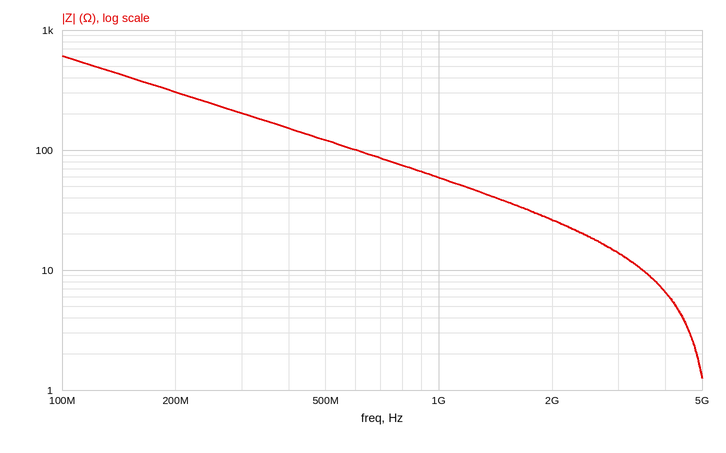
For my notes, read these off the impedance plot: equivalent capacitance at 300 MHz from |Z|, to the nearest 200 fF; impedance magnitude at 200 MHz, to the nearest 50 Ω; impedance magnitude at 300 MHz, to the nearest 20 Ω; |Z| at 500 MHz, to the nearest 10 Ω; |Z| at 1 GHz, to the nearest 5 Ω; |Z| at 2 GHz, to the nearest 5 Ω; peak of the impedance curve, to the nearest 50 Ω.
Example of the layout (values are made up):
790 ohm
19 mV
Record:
2.6 pF
300 Ω
200 Ω
120 Ω
60 Ω
25 Ω
600 Ω
